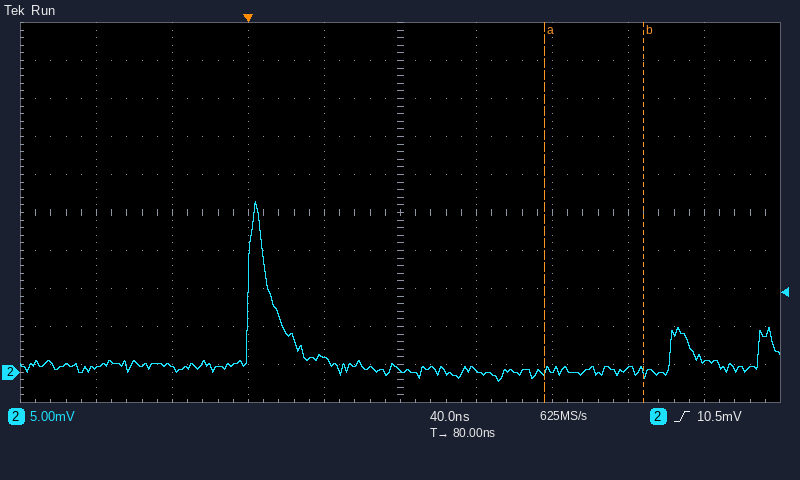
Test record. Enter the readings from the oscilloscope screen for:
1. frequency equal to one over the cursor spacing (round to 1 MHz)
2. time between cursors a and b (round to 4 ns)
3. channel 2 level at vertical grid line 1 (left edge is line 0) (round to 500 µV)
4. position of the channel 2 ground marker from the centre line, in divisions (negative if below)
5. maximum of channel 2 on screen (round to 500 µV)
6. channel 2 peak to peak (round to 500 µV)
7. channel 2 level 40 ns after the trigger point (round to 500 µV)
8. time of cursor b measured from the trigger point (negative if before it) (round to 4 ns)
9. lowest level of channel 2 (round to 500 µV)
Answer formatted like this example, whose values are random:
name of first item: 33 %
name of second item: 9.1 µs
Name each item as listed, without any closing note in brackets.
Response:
frequency equal to one over the cursor spacing: 19 MHz
time between cursors a and b: 52 ns
channel 2 level at vertical grid line 1 (left edge is line 0): 500 µV
position of the channel 2 ground marker from the centre line, in divisions: -4.2 div
maximum of channel 2 on screen: 22.5 mV
channel 2 peak to peak: 23.5 mV
channel 2 level 40 ns after the trigger point: 2.0 mV
time of cursor b measured from the trigger point (negative if before it): +208 ns
lowest level of channel 2: -1.0 mV
